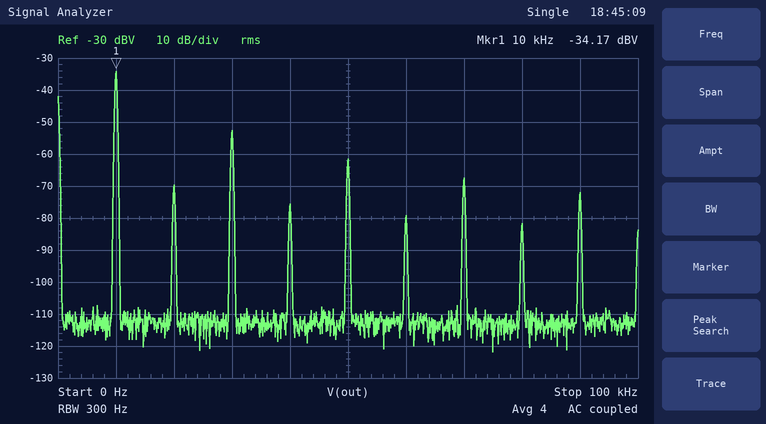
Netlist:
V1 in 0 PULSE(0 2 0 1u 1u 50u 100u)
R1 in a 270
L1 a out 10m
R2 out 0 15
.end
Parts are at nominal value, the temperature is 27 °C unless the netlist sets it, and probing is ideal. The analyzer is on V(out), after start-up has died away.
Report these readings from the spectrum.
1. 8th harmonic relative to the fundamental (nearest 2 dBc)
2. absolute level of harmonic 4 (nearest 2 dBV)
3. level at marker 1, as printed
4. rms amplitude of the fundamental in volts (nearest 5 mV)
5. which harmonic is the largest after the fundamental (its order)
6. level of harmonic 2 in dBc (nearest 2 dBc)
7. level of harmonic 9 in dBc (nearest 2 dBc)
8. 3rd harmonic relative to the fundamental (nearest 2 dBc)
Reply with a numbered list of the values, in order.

1. -48 dBc
2. -76 dBV
3. -34.17 dBV
4. 20 mV
5. 3
6. -36 dBc
7. -38 dBc
8. -18 dBc
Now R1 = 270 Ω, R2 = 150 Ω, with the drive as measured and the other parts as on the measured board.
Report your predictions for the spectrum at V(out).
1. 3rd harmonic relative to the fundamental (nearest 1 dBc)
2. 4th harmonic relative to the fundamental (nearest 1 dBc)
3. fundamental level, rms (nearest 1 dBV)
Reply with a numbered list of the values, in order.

1. -18 dBc
2. -41 dBc
3. -15 dBV
